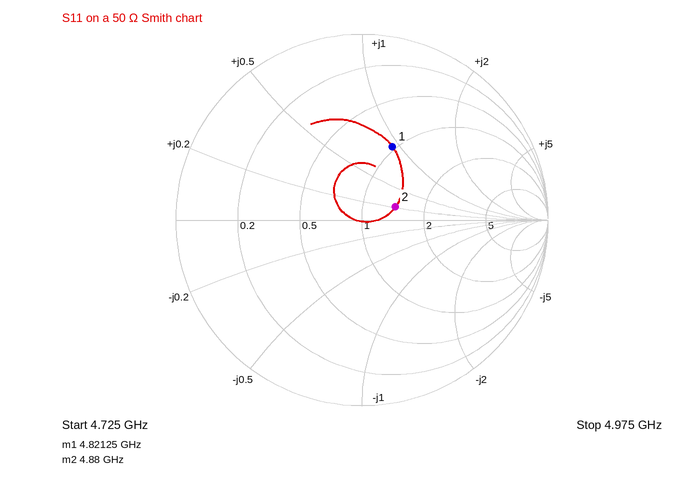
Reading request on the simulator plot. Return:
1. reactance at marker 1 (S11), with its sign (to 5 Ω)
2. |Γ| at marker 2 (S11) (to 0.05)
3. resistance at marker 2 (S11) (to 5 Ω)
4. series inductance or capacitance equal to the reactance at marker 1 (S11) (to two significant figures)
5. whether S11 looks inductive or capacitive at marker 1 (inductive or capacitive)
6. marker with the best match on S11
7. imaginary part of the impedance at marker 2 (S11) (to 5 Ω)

+45 Ω
0.20
70 Ω
1.5 nH
inductive
marker 2
+10 Ω
